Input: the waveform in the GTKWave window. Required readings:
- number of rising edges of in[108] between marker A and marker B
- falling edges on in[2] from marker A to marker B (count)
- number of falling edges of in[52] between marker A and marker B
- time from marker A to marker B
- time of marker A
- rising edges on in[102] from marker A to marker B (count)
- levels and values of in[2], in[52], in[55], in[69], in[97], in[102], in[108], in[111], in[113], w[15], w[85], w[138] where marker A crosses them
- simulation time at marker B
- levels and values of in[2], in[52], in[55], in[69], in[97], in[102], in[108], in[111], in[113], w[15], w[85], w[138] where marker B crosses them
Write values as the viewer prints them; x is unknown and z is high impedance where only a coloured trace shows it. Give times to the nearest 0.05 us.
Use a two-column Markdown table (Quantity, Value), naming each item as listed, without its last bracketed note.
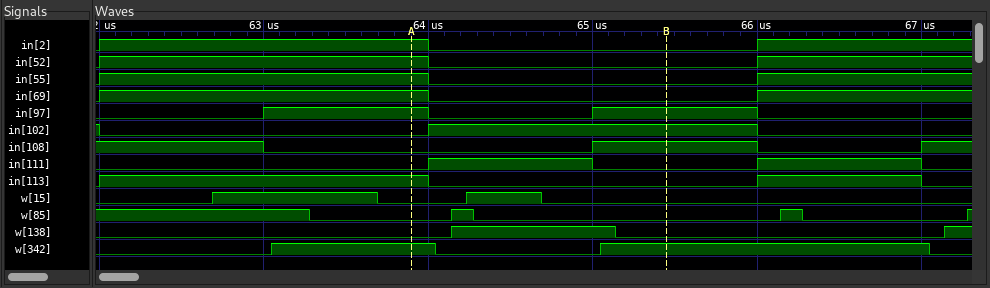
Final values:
| Quantity | Value |
|---|---|
| number of rising edges of in[108] between marker A and marker B | 1 |
| falling edges on in[2] from marker A to marker B | 1 |
| number of falling edges of in[52] between marker A and marker B | 1 |
| time from marker A to marker B | 1.55 us |
| time of marker A | 63.9 us |
| rising edges on in[102] from marker A to marker B | 1 |
| levels and values of in[2], in[52], in[55], in[69], in[97], in[102], in[108], in[111], in[113], w[15], w[85], w[138] where marker A crosses them | in[2]=1, in[52]=1, in[55]=1, in[69]=1, in[97]=1, in[102]=0, in[108]=0, in[111]=0, in[113]=1, w[15]=0, w[85]=0, w[138]=0 |
| simulation time at marker B | 65.45 us |
| levels and values of in[2], in[52], in[55], in[69], in[97], in[102], in[108], in[111], in[113], w[15], w[85], w[138] where marker B crosses them | in[2]=0, in[52]=0, in[55]=0, in[69]=0, in[97]=1, in[102]=1, in[108]=1, in[111]=0, in[113]=0, w[15]=0, w[85]=0, w[138]=0 |
